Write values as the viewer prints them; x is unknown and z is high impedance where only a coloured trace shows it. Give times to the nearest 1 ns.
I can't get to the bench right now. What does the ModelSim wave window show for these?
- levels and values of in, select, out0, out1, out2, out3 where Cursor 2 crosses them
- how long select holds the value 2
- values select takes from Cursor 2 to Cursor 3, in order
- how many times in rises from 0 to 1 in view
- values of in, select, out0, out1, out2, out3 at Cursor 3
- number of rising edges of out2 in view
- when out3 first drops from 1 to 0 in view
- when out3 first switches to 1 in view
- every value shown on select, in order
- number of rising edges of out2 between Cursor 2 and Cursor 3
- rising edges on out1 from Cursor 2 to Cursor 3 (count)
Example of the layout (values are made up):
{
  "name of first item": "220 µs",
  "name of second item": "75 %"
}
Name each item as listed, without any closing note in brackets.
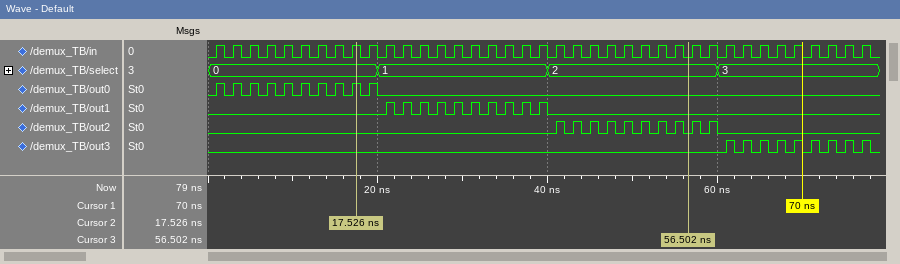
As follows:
{
  "levels and values of in, select, out0, out1, out2, out3 where Cursor 2 crosses them": "in=1, select=0, out0=1, out1=0, out2=0, out3=0",
  "how long select holds the value 2": "20 ns",
  "values select takes from Cursor 2 to Cursor 3, in order": "0, 1, 2",
  "how many times in rises from 0 to 1 in view": "39",
  "values of in, select, out0, out1, out2, out3 at Cursor 3": "in=0, select=2, out0=0, out1=0, out2=0, out3=0",
  "number of rising edges of out2 in view": "10",
  "when out3 first drops from 1 to 0 in view": "62 ns",
  "when out3 first switches to 1 in view": "61 ns",
  "every value shown on select, in order": "0, 1, 2, 3",
  "number of rising edges of out2 between Cursor 2 and Cursor 3": "8",
  "rising edges on out1 from Cursor 2 to Cursor 3": "10"
}
